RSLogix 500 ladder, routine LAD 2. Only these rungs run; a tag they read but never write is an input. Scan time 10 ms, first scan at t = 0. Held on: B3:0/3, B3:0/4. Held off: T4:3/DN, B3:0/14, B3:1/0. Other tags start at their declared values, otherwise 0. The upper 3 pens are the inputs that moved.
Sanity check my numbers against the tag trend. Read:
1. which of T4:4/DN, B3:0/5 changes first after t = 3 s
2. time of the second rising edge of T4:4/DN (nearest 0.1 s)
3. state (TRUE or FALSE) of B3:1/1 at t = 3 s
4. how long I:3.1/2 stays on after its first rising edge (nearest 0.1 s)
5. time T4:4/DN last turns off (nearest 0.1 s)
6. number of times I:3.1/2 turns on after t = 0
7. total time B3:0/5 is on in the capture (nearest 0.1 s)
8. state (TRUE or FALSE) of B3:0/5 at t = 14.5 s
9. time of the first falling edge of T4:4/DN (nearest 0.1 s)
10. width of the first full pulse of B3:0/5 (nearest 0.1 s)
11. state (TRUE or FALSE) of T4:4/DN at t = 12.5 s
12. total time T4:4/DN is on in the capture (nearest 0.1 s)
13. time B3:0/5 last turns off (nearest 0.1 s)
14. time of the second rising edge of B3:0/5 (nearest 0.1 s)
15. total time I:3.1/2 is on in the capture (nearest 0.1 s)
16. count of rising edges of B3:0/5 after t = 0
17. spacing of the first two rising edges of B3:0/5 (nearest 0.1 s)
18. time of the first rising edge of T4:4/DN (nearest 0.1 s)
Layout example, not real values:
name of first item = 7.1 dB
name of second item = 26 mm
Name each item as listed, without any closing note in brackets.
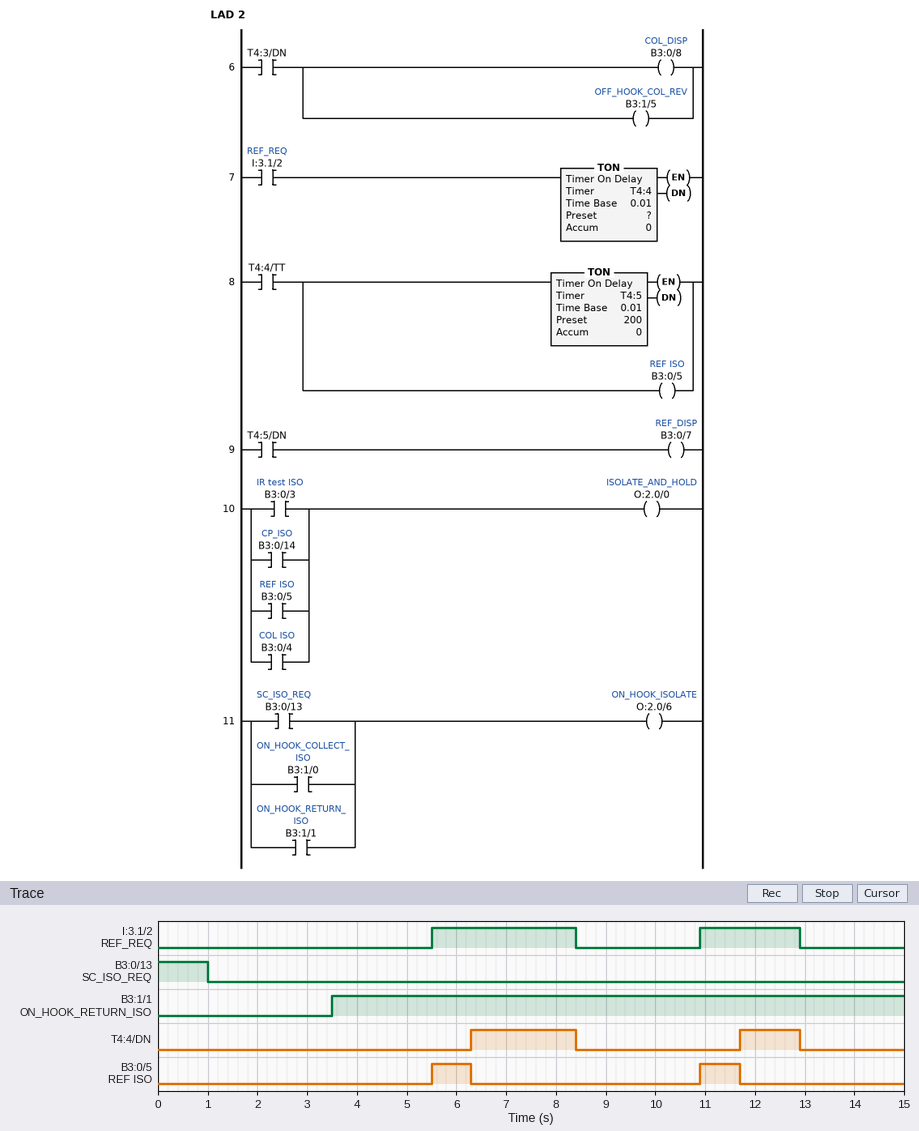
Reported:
which of T4:4/DN, B3:0/5 changes first after t = 3 s = B3:0/5
time of the second rising edge of T4:4/DN = 11.7 s
state (TRUE or FALSE) of B3:1/1 at t = 3 s = FALSE
how long I:3.1/2 stays on after its first rising edge = 2.9 s
time T4:4/DN last turns off = 12.9 s
number of times I:3.1/2 turns on after t = 0 = 2
total time B3:0/5 is on in the capture = 1.6 s
state (TRUE or FALSE) of B3:0/5 at t = 14.5 s = FALSE
time of the first falling edge of T4:4/DN = 8.4 s
width of the first full pulse of B3:0/5 = 0.8 s
state (TRUE or FALSE) of T4:4/DN at t = 12.5 s = TRUE
total time T4:4/DN is on in the capture = 3.3 s
time B3:0/5 last turns off = 11.7 s
time of the second rising edge of B3:0/5 = 10.9 s
total time I:3.1/2 is on in the capture = 4.9 s
count of rising edges of B3:0/5 after t = 0 = 2
spacing of the first two rising edges of B3:0/5 = 5.4 s
time of the first rising edge of T4:4/DN = 6.3 s
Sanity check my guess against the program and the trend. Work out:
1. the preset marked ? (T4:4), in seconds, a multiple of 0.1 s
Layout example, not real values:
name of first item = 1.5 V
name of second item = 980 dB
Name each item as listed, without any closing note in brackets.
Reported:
the preset marked ? (T4:4), in seconds, a multiple of 0.1 s = 0.8 s
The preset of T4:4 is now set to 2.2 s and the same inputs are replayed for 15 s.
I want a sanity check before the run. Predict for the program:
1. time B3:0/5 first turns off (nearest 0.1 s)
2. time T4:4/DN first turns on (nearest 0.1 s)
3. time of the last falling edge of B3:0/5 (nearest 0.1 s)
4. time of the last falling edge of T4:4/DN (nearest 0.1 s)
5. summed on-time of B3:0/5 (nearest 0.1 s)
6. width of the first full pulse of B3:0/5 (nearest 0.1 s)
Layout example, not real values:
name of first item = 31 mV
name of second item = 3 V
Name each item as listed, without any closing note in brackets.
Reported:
time B3:0/5 first turns off = 7.7 s
time T4:4/DN first turns on = 7.7 s
time of the last falling edge of B3:0/5 = 12.9 s
time of the last falling edge of T4:4/DN = 8.4 s
summed on-time of B3:0/5 = 4.2 s
width of the first full pulse of B3:0/5 = 2.2 s
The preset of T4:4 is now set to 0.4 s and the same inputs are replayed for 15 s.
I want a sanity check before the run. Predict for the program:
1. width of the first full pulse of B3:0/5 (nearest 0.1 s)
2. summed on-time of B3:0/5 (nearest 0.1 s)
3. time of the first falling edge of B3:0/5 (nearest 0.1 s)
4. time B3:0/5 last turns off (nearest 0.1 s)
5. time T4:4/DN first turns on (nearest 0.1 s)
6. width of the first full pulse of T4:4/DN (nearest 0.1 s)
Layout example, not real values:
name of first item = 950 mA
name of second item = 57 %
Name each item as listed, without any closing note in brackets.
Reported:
width of the first full pulse of B3:0/5 = 0.4 s
summed on-time of B3:0/5 = 0.8 s
time of the first falling edge of B3:0/5 = 5.9 s
time B3:0/5 last turns off = 11.3 s
time T4:4/DN first turns on = 5.9 s
width of the first full pulse of T4:4/DN = 2.5 s
